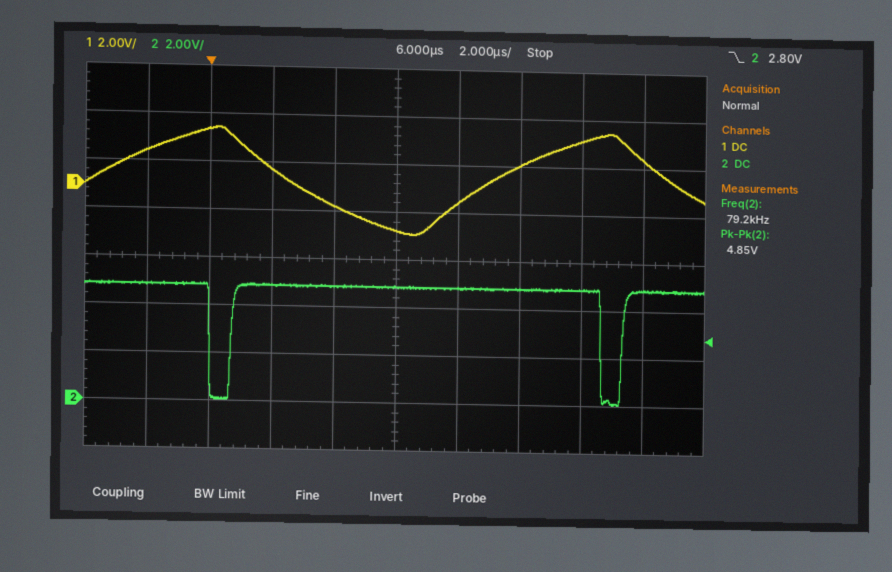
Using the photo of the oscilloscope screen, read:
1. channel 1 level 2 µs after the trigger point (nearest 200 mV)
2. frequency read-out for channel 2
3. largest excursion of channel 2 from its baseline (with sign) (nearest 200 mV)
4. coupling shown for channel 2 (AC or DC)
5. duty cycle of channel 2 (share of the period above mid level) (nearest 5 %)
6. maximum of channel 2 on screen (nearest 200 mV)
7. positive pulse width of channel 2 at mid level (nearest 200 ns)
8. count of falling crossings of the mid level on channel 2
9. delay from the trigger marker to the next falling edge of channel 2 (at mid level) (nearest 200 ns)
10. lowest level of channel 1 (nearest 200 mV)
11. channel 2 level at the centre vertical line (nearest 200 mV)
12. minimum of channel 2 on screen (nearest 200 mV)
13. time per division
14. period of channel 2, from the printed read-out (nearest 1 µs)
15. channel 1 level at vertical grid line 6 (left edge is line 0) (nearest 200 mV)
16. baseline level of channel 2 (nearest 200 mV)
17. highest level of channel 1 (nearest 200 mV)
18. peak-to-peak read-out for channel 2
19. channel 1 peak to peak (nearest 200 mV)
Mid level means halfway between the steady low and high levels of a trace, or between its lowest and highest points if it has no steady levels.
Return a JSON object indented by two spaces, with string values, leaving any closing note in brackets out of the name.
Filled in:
{
  "channel 1 level 2 µs after the trigger point": "800 mV",
  "frequency read-out for channel 2": "79.2 kHz",
  "largest excursion of channel 2 from its baseline (with sign)": "-4.8 V",
  "coupling shown for channel 2": "DC",
  "duty cycle of channel 2 (share of the period above mid level)": "95 %",
  "maximum of channel 2 on screen": "5.0 V",
  "positive pulse width of channel 2 at mid level": "12.0 µs",
  "count of falling crossings of the mid level on channel 2": "2",
  "delay from the trigger marker to the next falling edge of channel 2 (at mid level)": "12.6 µs",
  "lowest level of channel 1": "-2.0 V",
  "channel 2 level at the centre vertical line": "4.8 V",
  "minimum of channel 2 on screen": "0.0 V",
  "time per division": "2 µs",
  "period of channel 2, from the printed read-out": "13 µs",
  "channel 1 level at vertical grid line 6 (left edge is line 0)": "-600 mV",
  "baseline level of channel 2": "4.8 V",
  "highest level of channel 1": "2.4 V",
  "peak-to-peak read-out for channel 2": "4.85 V",
  "channel 1 peak to peak": "4.4 V"
}
